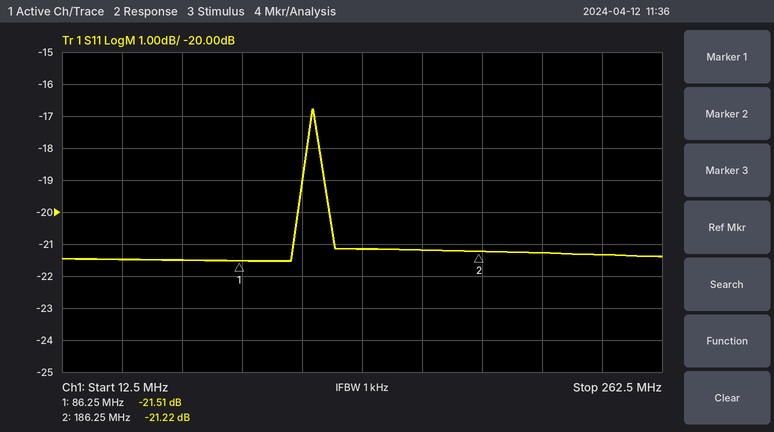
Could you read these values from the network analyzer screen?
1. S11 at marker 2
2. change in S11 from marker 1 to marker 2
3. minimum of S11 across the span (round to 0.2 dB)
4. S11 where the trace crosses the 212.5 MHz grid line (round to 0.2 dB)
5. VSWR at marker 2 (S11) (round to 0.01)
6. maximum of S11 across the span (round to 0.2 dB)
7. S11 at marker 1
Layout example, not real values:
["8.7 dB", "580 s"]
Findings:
["-21.22 dB", "0.29 dB", "-21.6 dB", "-21.2 dB", "1.19", "-16.8 dB", "-21.51 dB"]
